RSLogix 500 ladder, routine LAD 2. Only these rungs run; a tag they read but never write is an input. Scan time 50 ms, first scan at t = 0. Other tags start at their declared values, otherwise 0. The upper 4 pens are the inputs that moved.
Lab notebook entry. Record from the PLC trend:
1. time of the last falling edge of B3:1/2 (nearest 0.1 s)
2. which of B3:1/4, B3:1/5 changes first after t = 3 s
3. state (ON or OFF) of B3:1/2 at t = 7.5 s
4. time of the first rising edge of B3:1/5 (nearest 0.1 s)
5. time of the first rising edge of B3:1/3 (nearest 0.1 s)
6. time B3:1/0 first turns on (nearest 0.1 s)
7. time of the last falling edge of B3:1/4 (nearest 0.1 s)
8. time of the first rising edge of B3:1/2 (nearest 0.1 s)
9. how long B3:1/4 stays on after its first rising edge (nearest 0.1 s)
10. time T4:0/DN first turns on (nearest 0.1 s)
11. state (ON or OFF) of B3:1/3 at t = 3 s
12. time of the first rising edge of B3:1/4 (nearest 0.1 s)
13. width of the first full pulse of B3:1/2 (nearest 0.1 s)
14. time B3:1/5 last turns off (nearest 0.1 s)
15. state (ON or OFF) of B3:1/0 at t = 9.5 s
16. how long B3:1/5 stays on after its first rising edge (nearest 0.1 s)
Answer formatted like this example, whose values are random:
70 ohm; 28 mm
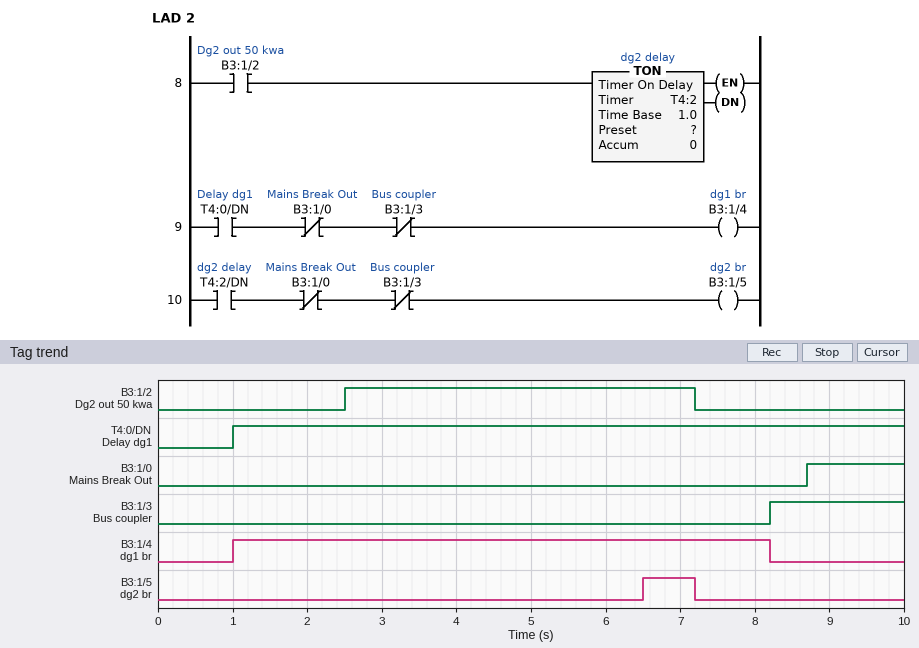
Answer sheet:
7.2 s; B3:1/5; OFF; 6.5 s; 8.2 s; 8.7 s; 8.2 s; 2.5 s; 7.2 s; 1.0 s; OFF; 1.0 s; 4.7 s; 7.2 s; ON; 0.7 s
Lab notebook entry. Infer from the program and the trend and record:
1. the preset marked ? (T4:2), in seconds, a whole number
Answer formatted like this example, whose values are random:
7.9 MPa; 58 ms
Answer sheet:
4 s
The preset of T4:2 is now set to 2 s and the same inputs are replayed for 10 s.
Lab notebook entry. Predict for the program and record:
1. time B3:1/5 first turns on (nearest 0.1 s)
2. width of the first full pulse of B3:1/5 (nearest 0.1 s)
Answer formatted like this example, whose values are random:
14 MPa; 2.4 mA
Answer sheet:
4.5 s; 2.7 s
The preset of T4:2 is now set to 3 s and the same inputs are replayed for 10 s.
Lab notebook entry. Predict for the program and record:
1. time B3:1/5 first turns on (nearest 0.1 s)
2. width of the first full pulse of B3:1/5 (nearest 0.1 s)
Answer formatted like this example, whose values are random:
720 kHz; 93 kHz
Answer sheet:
5.5 s; 1.7 s
